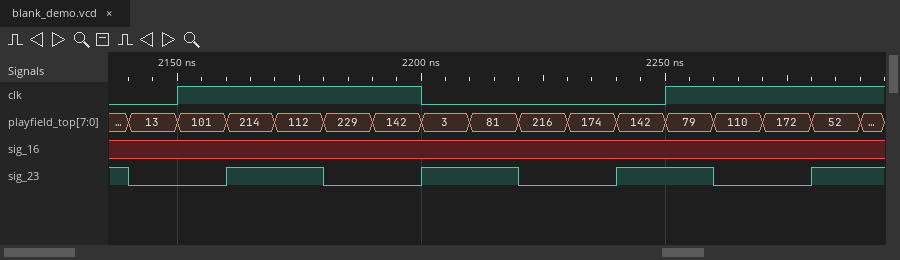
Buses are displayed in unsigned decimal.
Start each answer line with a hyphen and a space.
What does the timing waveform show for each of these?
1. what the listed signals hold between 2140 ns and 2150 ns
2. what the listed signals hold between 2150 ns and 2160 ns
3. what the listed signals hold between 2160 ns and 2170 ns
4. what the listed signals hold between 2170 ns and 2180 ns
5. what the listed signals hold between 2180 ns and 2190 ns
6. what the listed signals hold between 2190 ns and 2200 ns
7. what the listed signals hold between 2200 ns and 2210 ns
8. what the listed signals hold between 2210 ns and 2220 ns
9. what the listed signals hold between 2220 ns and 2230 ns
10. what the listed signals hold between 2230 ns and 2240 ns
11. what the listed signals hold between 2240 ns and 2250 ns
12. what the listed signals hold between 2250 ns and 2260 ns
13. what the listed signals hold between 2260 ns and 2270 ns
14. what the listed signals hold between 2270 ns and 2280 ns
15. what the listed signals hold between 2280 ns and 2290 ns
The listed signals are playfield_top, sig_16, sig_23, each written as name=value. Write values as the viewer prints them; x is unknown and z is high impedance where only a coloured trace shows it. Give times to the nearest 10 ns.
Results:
- playfield_top=13, sig_16=x, sig_23=0
- playfield_top=101, sig_16=x, sig_23=0
- playfield_top=214, sig_16=x, sig_23=1
- playfield_top=112, sig_16=x, sig_23=1
- playfield_top=229, sig_16=x, sig_23=0
- playfield_top=142, sig_16=x, sig_23=0
- playfield_top=3, sig_16=x, sig_23=1
- playfield_top=81, sig_16=x, sig_23=1
- playfield_top=216, sig_16=x, sig_23=0
- playfield_top=174, sig_16=x, sig_23=0
- playfield_top=142, sig_16=x, sig_23=1
- playfield_top=79, sig_16=x, sig_23=1
- playfield_top=110, sig_16=x, sig_23=0
- playfield_top=172, sig_16=x, sig_23=0
- playfield_top=52, sig_16=x, sig_23=1
